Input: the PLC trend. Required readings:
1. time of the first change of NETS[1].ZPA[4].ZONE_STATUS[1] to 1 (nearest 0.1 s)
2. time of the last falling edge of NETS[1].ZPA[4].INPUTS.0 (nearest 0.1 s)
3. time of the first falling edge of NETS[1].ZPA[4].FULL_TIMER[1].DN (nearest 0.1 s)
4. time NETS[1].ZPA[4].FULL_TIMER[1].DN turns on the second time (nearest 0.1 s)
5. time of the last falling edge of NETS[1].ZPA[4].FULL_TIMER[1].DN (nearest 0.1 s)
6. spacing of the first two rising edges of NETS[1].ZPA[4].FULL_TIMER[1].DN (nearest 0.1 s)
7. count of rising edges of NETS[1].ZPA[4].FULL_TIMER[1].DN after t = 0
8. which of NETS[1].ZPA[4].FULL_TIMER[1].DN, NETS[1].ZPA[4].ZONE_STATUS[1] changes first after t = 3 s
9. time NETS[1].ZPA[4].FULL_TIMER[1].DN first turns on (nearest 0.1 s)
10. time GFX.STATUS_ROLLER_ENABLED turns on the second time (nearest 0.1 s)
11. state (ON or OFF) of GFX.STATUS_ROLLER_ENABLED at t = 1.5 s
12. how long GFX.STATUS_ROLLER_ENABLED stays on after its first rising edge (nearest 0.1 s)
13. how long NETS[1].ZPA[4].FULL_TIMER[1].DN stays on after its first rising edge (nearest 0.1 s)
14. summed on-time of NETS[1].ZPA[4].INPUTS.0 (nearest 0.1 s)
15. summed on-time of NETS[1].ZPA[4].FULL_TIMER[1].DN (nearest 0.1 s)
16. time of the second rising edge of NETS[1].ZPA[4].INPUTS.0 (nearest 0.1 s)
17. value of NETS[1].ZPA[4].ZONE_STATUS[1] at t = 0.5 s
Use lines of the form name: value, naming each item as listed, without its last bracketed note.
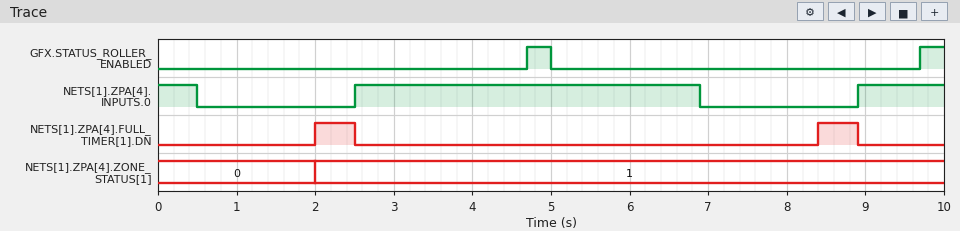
time of the first change of NETS[1].ZPA[4].ZONE_STATUS[1] to 1: 2.0 s
time of the last falling edge of NETS[1].ZPA[4].INPUTS.0: 6.9 s
time of the first falling edge of NETS[1].ZPA[4].FULL_TIMER[1].DN: 2.5 s
time NETS[1].ZPA[4].FULL_TIMER[1].DN turns on the second time: 8.4 s
time of the last falling edge of NETS[1].ZPA[4].FULL_TIMER[1].DN: 8.9 s
spacing of the first two rising edges of NETS[1].ZPA[4].FULL_TIMER[1].DN: 6.4 s
count of rising edges of NETS[1].ZPA[4].FULL_TIMER[1].DN after t = 0: 2
which of NETS[1].ZPA[4].FULL_TIMER[1].DN, NETS[1].ZPA[4].ZONE_STATUS[1] changes first after t = 3 s: NETS[1].ZPA[4].FULL_TIMER[1].DN
time NETS[1].ZPA[4].FULL_TIMER[1].DN first turns on: 2.0 s
time GFX.STATUS_ROLLER_ENABLED turns on the second time: 9.7 s
state (ON or OFF) of GFX.STATUS_ROLLER_ENABLED at t = 1.5 s: OFF
how long GFX.STATUS_ROLLER_ENABLED stays on after its first rising edge: 0.3 s
how long NETS[1].ZPA[4].FULL_TIMER[1].DN stays on after its first rising edge: 0.5 s
summed on-time of NETS[1].ZPA[4].INPUTS.0: 6.0 s
summed on-time of NETS[1].ZPA[4].FULL_TIMER[1].DN: 1.0 s
time of the second rising edge of NETS[1].ZPA[4].INPUTS.0: 8.9 s
value of NETS[1].ZPA[4].ZONE_STATUS[1] at t = 0.5 s: 0
